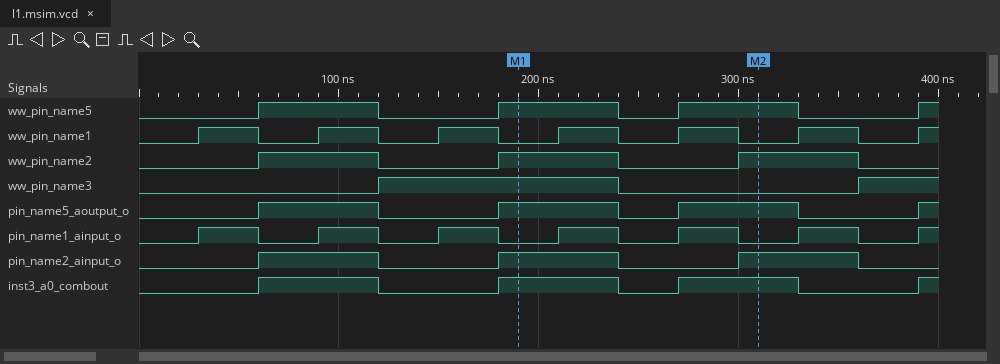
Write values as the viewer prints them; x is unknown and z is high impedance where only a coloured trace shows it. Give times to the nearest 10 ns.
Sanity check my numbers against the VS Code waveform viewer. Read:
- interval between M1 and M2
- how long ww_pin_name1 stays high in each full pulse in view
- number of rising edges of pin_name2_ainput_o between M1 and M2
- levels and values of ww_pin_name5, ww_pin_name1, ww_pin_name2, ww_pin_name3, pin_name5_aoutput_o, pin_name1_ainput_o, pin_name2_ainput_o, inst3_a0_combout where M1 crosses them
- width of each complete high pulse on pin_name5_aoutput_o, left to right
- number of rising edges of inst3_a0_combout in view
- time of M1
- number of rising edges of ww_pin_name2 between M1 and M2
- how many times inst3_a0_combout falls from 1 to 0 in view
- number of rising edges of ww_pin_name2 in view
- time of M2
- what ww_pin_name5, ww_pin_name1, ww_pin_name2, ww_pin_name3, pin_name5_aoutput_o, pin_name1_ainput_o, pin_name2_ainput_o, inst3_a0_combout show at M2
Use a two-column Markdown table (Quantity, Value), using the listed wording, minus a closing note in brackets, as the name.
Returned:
| Quantity | Value |
|---|---|
| interval between M1 and M2 | 120 ns |
| how long ww_pin_name1 stays high in each full pulse in view | 30 ns, 30 ns, 30 ns, 30 ns, 30 ns, 30 ns |
| number of rising edges of pin_name2_ainput_o between M1 and M2 | 1 |
| levels and values of ww_pin_name5, ww_pin_name1, ww_pin_name2, ww_pin_name3, pin_name5_aoutput_o, pin_name1_ainput_o, pin_name2_ainput_o, inst3_a0_combout where M1 crosses them | ww_pin_name5=1, ww_pin_name1=0, ww_pin_name2=1, ww_pin_name3=1, pin_name5_aoutput_o=1, pin_name1_ainput_o=0, pin_name2_ainput_o=1, inst3_a0_combout=1 |
| width of each complete high pulse on pin_name5_aoutput_o, left to right | 60 ns, 60 ns, 60 ns |
| number of rising edges of inst3_a0_combout in view | 4 |
| time of M1 | 190 ns |
| number of rising edges of ww_pin_name2 between M1 and M2 | 1 |
| how many times inst3_a0_combout falls from 1 to 0 in view | 3 |
| number of rising edges of ww_pin_name2 in view | 3 |
| time of M2 | 310 ns |
| what ww_pin_name5, ww_pin_name1, ww_pin_name2, ww_pin_name3, pin_name5_aoutput_o, pin_name1_ainput_o, pin_name2_ainput_o, inst3_a0_combout show at M2 | ww_pin_name5=1, ww_pin_name1=0, ww_pin_name2=1, ww_pin_name3=0, pin_name5_aoutput_o=1, pin_name1_ainput_o=0, pin_name2_ainput_o=1, inst3_a0_combout=1 |
